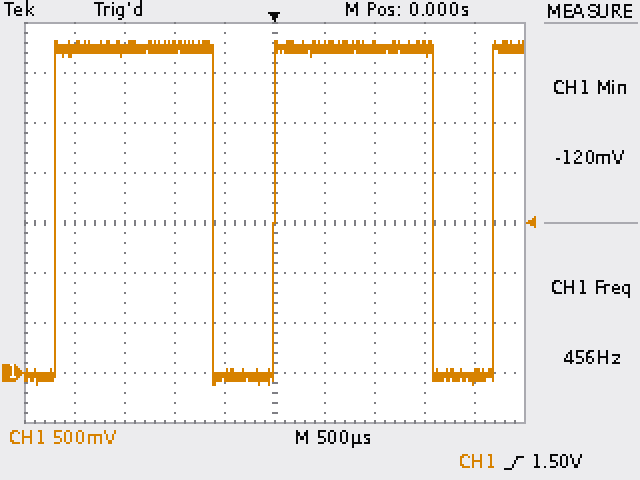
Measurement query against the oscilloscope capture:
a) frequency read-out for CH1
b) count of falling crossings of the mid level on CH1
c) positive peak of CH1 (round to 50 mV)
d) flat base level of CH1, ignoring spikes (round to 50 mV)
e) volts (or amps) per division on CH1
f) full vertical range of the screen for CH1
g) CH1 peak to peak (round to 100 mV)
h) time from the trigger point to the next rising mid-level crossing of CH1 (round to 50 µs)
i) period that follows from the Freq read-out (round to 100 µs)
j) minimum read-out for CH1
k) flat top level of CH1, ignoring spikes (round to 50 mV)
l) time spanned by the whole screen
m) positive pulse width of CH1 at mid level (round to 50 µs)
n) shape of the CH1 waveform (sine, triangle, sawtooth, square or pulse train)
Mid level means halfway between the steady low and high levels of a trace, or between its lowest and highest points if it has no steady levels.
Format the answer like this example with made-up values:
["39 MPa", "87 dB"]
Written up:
["456 Hz", "2", "3.30 V", "-50 mV", "500 mV", "4 V", "3.40 V", "2.20 ms", "2.2 ms", "-120 mV", "3.25 V", "5 ms", "1.60 ms", "pulse train"]
